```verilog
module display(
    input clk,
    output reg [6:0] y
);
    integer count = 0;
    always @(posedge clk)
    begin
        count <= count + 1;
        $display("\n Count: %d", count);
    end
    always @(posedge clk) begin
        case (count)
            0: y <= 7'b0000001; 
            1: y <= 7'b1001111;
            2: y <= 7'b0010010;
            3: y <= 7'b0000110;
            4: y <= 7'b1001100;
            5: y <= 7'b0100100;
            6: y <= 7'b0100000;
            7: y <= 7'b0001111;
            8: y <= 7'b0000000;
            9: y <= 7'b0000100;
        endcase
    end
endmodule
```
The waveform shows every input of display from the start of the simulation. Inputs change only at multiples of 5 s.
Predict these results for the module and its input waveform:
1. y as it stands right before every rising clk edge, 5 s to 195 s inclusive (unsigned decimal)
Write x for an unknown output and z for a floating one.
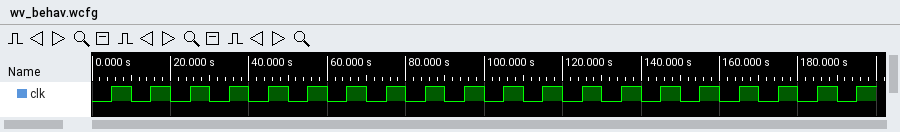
x, 1, 79, 18, 6, 76, 36, 32, 15, 0, 4, 4, 4, 4, 4, 4, 4, 4, 4, 4
